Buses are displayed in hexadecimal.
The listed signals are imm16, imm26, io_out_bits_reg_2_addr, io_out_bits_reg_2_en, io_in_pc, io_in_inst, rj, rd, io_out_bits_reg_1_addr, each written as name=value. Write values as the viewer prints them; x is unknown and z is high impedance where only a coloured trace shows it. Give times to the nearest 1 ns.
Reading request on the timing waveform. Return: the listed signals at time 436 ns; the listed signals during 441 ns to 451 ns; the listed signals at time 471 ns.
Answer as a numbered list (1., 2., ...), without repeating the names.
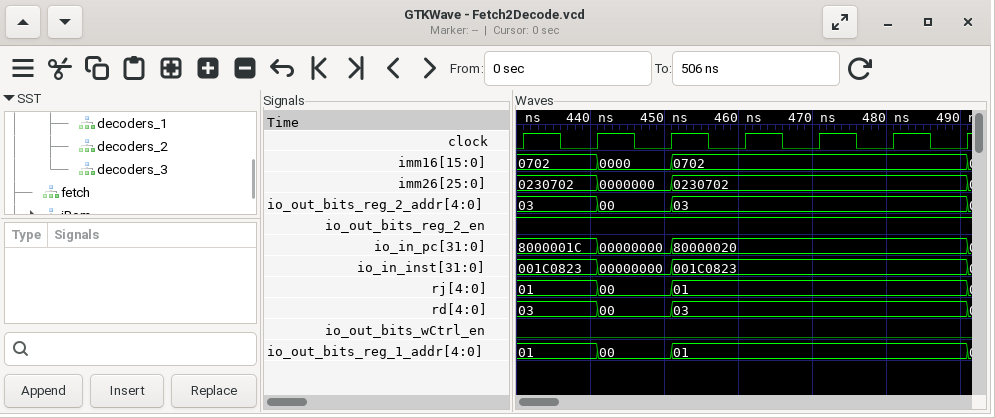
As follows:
1. imm16=0702, imm26=0230702, io_out_bits_reg_2_addr=03, io_out_bits_reg_2_en=1, io_in_pc=8000001C, io_in_inst=001C0823, rj=01, rd=03, io_out_bits_reg_1_addr=01
2. imm16=0000, imm26=0000000, io_out_bits_reg_2_addr=00, io_out_bits_reg_2_en=1, io_in_pc=00000000, io_in_inst=00000000, rj=00, rd=00, io_out_bits_reg_1_addr=00
3. imm16=0702, imm26=0230702, io_out_bits_reg_2_addr=03, io_out_bits_reg_2_en=1, io_in_pc=80000020, io_in_inst=001C0823, rj=01, rd=03, io_out_bits_reg_1_addr=01
